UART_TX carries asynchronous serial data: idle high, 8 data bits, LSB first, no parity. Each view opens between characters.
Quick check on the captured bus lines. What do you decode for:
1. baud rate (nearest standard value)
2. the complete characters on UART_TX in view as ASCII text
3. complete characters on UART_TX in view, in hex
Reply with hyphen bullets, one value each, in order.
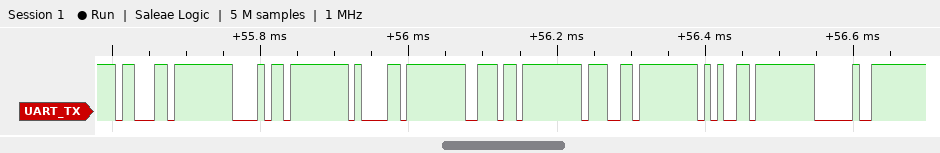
- 115200 baud
- "change "
- 63, 68, 61, 6E, 67, 65, 20
